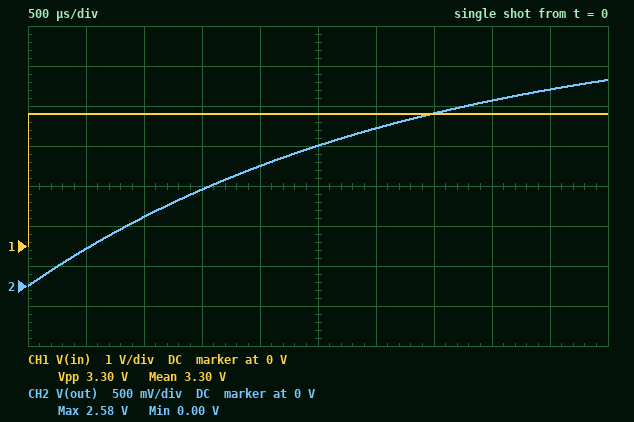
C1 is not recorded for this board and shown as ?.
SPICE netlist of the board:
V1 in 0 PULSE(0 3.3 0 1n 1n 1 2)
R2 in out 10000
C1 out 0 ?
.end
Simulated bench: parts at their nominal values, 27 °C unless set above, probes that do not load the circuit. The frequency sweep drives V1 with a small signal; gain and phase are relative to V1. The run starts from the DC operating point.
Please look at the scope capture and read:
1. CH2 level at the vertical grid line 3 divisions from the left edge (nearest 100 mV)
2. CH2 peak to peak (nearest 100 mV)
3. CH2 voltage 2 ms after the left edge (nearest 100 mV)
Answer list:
1.2 V
2.6 V
1.5 V
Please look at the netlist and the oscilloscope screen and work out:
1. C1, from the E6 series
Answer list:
330 nF
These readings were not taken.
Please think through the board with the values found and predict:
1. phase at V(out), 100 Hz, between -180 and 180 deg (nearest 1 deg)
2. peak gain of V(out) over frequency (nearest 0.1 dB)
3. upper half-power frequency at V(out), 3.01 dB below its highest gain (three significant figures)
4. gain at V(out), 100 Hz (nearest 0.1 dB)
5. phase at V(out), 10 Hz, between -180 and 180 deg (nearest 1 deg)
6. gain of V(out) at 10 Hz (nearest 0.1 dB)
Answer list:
-64 deg
0 dB
48.2 Hz
-7.2 dB
-12 deg
-0.2 dB
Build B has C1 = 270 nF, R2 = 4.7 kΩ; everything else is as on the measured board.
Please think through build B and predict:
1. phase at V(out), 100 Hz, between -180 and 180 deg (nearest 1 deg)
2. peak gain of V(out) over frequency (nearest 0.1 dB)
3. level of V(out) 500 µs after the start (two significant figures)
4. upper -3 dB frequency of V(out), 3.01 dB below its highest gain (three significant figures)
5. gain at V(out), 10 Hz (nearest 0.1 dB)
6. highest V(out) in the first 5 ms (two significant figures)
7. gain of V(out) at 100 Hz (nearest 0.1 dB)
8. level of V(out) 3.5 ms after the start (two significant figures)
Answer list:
-39 deg
0 dB
1.1 V
125 Hz
0 dB
3.2 V
-2.1 dB
3.1 V
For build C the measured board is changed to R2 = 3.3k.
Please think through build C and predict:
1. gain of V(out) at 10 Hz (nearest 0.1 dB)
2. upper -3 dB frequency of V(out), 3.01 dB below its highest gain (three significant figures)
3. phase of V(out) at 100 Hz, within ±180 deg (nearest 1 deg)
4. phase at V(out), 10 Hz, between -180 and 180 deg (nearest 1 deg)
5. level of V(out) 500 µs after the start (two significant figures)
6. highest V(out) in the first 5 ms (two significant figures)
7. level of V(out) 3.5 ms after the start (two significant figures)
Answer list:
0 dB
146 Hz
-34 deg
-4 deg
1.2 V
3.3 V
3.2 V
